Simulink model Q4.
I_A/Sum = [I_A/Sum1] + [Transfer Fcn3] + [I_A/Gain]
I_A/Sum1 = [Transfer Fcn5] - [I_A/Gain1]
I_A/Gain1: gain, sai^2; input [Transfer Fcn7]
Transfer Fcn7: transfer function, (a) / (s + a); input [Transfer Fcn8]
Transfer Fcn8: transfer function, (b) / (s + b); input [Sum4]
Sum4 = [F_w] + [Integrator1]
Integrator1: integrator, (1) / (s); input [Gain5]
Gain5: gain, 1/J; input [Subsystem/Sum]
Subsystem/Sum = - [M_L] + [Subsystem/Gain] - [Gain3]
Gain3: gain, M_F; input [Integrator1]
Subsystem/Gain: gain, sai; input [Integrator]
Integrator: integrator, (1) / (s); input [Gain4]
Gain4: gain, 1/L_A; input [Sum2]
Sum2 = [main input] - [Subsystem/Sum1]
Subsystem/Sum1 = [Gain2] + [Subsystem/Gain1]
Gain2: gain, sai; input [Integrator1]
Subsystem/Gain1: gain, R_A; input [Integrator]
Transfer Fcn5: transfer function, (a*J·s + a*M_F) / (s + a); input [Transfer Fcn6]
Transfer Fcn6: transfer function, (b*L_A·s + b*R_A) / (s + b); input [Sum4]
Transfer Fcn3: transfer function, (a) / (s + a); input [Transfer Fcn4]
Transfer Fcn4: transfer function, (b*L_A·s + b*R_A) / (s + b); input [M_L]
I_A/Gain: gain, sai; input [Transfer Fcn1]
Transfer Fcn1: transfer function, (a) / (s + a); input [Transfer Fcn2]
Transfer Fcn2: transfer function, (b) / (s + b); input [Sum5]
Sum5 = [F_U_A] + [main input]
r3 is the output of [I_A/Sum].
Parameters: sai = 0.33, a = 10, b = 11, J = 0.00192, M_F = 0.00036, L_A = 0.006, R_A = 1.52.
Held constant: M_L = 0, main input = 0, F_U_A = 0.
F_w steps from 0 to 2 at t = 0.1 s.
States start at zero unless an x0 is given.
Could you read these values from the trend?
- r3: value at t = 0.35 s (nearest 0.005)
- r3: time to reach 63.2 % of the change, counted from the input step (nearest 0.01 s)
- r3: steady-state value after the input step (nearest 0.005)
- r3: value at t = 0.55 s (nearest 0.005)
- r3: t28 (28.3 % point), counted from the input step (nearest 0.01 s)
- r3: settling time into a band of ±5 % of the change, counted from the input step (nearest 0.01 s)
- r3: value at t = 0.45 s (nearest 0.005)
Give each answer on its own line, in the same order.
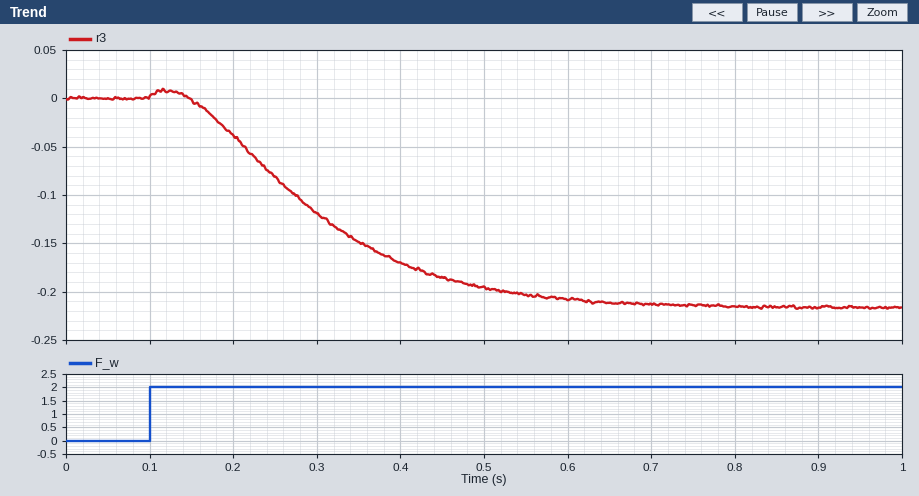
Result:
-0.150
0.23 s
-0.215
-0.205
0.13 s
0.48 s
-0.185
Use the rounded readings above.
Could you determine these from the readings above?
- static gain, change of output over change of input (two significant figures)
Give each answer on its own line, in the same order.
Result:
-0.11
